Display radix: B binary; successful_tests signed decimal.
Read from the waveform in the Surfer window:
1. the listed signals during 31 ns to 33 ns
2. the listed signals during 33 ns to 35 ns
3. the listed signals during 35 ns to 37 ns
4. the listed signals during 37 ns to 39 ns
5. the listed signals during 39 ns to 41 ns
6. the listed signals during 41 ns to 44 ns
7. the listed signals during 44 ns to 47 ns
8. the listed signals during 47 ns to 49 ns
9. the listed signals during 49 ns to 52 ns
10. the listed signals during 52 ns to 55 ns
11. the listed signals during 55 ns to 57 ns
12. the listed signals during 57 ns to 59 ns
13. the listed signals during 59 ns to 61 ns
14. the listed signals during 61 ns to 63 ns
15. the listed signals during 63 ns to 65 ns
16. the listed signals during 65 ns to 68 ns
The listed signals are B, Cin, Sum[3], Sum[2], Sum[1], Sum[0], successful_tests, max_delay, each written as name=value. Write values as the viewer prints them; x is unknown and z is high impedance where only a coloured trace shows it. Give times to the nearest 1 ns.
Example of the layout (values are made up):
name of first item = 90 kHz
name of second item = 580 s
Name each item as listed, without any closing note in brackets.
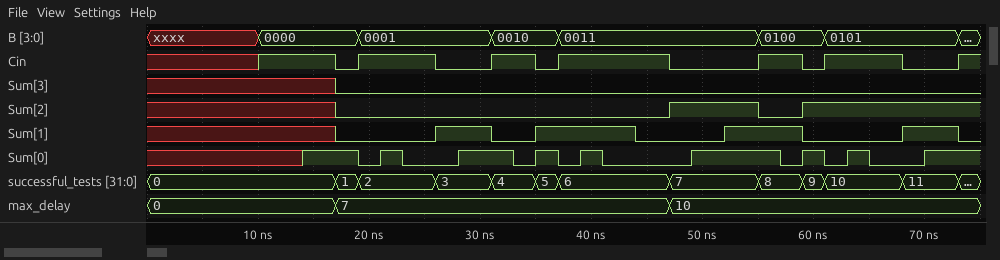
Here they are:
the listed signals during 31 ns to 33 ns = B=0010, Cin=1, Sum[3]=0, Sum[2]=0, Sum[1]=0, Sum[0]=1, successful_tests=4, max_delay=7
the listed signals during 33 ns to 35 ns = B=0010, Cin=1, Sum[3]=0, Sum[2]=0, Sum[1]=0, Sum[0]=0, successful_tests=4, max_delay=7
the listed signals during 35 ns to 37 ns = B=0010, Cin=0, Sum[3]=0, Sum[2]=0, Sum[1]=1, Sum[0]=1, successful_tests=5, max_delay=7
the listed signals during 37 ns to 39 ns = B=0011, Cin=1, Sum[3]=0, Sum[2]=0, Sum[1]=1, Sum[0]=0, successful_tests=6, max_delay=7
the listed signals during 39 ns to 41 ns = B=0011, Cin=1, Sum[3]=0, Sum[2]=0, Sum[1]=1, Sum[0]=1, successful_tests=6, max_delay=7
the listed signals during 41 ns to 44 ns = B=0011, Cin=1, Sum[3]=0, Sum[2]=0, Sum[1]=1, Sum[0]=0, successful_tests=6, max_delay=7
the listed signals during 44 ns to 47 ns = B=0011, Cin=1, Sum[3]=0, Sum[2]=0, Sum[1]=0, Sum[0]=0, successful_tests=6, max_delay=7
the listed signals during 47 ns to 49 ns = B=0011, Cin=0, Sum[3]=0, Sum[2]=1, Sum[1]=0, Sum[0]=0, successful_tests=7, max_delay=10
the listed signals during 49 ns to 52 ns = B=0011, Cin=0, Sum[3]=0, Sum[2]=1, Sum[1]=0, Sum[0]=1, successful_tests=7, max_delay=10
the listed signals during 52 ns to 55 ns = B=0011, Cin=0, Sum[3]=0, Sum[2]=1, Sum[1]=1, Sum[0]=1, successful_tests=7, max_delay=10
the listed signals during 55 ns to 57 ns = B=0100, Cin=1, Sum[3]=0, Sum[2]=0, Sum[1]=1, Sum[0]=1, successful_tests=8, max_delay=10
the listed signals during 57 ns to 59 ns = B=0100, Cin=1, Sum[3]=0, Sum[2]=0, Sum[1]=1, Sum[0]=0, successful_tests=8, max_delay=10
the listed signals during 59 ns to 61 ns = B=0100, Cin=0, Sum[3]=0, Sum[2]=1, Sum[1]=0, Sum[0]=1, successful_tests=9, max_delay=10
the listed signals during 61 ns to 63 ns = B=0101, Cin=1, Sum[3]=0, Sum[2]=1, Sum[1]=0, Sum[0]=0, successful_tests=10, max_delay=10
the listed signals during 63 ns to 65 ns = B=0101, Cin=1, Sum[3]=0, Sum[2]=1, Sum[1]=0, Sum[0]=1, successful_tests=10, max_delay=10
the listed signals during 65 ns to 68 ns = B=0101, Cin=1, Sum[3]=0, Sum[2]=1, Sum[1]=0, Sum[0]=0, successful_tests=10, max_delay=10
